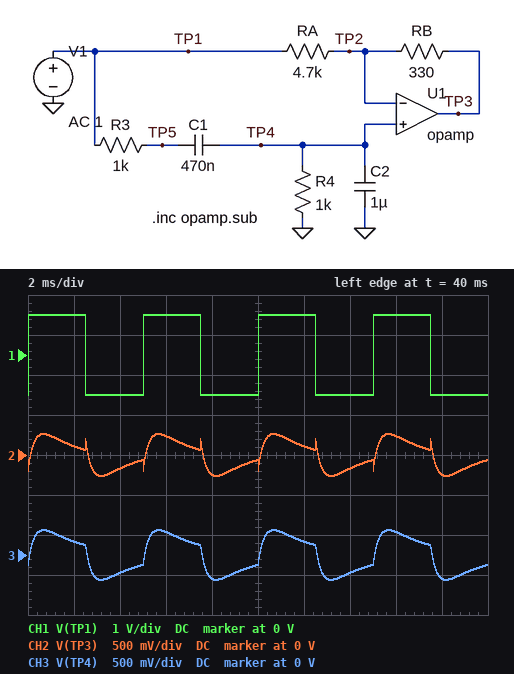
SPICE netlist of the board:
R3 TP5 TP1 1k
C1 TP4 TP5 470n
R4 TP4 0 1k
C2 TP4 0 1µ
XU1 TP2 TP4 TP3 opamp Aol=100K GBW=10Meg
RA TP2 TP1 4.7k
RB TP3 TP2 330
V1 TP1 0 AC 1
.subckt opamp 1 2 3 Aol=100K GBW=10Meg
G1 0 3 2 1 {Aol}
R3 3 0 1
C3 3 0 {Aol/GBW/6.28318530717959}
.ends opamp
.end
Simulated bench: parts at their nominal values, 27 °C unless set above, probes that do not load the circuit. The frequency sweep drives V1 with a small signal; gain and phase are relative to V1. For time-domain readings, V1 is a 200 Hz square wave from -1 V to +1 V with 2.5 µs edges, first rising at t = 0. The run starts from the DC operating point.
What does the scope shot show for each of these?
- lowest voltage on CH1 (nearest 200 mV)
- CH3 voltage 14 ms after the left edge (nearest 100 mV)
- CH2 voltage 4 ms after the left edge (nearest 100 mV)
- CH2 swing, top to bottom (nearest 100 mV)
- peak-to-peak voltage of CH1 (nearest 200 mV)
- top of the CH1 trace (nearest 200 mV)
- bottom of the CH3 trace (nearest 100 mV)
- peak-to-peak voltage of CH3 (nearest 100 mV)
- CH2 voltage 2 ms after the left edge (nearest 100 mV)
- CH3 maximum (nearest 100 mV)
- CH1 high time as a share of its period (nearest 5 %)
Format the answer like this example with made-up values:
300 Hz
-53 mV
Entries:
-1.0 V
-200 mV
-200 mV
500 mV
2.0 V
1.0 V
-300 mV
600 mV
100 mV
300 mV
50 %
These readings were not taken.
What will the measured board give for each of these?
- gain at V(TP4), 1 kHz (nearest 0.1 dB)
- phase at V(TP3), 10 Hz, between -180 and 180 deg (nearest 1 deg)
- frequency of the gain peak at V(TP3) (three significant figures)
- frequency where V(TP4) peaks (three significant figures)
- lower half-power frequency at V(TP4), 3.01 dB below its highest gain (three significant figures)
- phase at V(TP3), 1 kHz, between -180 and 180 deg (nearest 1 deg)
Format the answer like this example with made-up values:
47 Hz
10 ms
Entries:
-17.2 dB
155 deg
232 Hz
232 Hz
73.8 Hz
-83 deg
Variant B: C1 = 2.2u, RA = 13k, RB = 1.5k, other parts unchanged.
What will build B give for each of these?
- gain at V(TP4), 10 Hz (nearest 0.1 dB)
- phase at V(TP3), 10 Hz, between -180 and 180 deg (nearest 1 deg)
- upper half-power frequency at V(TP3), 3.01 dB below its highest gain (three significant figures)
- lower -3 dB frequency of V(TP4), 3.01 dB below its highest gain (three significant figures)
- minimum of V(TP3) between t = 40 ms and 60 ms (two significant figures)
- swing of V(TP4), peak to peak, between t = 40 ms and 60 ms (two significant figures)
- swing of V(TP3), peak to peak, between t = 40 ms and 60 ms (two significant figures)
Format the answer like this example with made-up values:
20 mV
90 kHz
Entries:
-17.6 dB
116 deg
470 Hz
27.5 Hz
-520 mV
830 mV
1.0 V
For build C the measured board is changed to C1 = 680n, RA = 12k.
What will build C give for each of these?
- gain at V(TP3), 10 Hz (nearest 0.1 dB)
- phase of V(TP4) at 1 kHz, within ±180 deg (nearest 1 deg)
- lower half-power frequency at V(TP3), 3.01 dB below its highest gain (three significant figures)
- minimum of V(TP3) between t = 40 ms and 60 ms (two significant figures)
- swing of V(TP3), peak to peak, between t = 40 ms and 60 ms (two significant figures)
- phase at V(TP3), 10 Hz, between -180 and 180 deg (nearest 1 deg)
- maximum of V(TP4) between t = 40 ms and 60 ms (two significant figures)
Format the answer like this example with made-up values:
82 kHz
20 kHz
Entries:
-26.4 dB
-60 deg
60.2 Hz
-330 mV
660 mV
116 deg
350 mV
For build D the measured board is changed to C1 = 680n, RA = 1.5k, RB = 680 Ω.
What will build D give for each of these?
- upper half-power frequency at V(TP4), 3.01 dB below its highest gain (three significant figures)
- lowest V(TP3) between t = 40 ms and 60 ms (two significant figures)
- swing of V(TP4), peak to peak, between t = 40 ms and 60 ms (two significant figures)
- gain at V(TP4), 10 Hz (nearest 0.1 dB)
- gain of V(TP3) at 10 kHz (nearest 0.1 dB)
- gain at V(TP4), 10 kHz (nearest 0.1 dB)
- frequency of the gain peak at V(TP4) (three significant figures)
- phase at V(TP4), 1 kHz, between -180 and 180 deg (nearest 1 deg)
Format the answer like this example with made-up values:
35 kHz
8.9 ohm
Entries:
613 Hz
-710 mV
690 mV
-27.5 dB
-6.9 dB
-36.0 dB
193 Hz
-60 deg
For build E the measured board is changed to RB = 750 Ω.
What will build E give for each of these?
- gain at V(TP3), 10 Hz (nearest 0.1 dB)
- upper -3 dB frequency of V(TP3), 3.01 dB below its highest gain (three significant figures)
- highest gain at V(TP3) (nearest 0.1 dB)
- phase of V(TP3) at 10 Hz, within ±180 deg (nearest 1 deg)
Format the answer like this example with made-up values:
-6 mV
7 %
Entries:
-16.0 dB
8.62 MHz
-15.9 dB
168 deg
